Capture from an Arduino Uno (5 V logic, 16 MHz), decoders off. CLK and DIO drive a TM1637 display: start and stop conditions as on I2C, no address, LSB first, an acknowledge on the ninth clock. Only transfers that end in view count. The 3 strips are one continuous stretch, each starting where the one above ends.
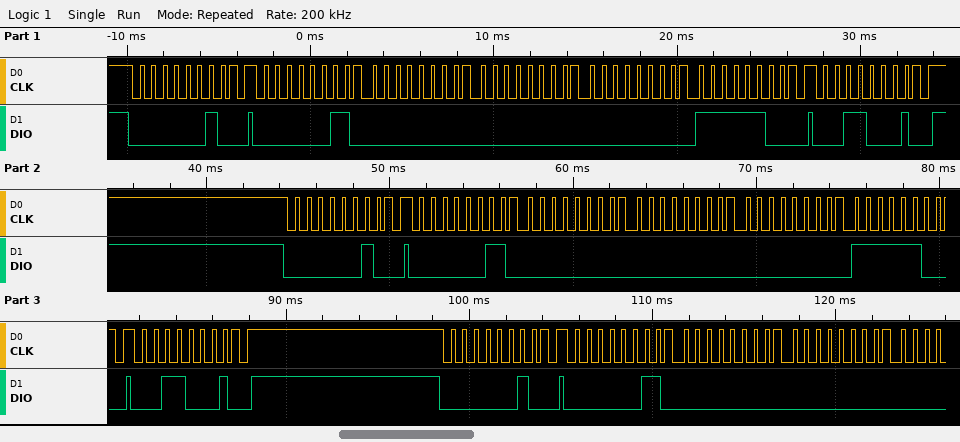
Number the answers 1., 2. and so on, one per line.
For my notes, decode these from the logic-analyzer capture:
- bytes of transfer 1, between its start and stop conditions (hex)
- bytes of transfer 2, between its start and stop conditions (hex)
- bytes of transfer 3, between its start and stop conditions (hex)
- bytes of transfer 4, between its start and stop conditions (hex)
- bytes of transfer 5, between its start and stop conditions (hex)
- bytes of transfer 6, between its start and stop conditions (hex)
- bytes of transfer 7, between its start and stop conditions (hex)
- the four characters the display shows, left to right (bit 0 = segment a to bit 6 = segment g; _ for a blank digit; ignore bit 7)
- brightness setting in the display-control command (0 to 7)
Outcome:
1. 40
2. C0 00 00 00 3F
3. 8C
4. 40
5. C0 00 00 00 3F
6. 8C
7. 40
8. ___0
9. 4
